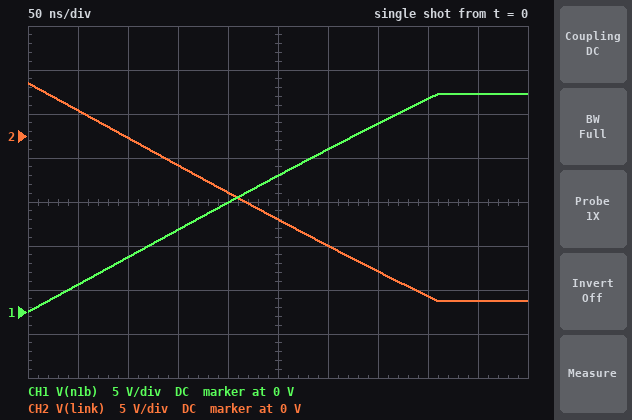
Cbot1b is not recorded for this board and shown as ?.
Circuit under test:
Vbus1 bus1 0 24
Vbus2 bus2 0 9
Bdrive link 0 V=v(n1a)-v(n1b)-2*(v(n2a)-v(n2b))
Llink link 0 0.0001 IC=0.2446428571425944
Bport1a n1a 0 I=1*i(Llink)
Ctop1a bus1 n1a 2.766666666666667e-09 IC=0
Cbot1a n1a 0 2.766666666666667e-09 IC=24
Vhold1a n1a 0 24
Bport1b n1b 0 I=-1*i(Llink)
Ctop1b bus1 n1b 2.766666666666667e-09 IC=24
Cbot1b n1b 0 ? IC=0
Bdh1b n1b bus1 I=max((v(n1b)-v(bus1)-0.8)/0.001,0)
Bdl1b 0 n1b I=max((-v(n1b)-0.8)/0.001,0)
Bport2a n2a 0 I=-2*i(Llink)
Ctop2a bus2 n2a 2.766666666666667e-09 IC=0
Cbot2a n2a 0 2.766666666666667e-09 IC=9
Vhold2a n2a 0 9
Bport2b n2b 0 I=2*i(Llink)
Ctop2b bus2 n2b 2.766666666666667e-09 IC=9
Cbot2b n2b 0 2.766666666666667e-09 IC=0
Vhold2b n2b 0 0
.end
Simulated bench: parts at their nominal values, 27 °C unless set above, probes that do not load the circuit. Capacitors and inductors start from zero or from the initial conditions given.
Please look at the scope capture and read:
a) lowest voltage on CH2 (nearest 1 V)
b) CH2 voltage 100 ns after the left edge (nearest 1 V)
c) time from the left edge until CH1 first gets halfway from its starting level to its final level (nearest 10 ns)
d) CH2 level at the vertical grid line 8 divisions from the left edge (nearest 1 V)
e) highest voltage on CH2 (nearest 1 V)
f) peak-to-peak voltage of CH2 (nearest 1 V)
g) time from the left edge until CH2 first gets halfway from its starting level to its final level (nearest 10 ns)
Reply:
-19 V
0 V
200 ns
-18 V
6 V
25 V
200 ns
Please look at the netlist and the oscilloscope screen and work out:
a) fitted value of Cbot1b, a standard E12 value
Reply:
1.2 nF
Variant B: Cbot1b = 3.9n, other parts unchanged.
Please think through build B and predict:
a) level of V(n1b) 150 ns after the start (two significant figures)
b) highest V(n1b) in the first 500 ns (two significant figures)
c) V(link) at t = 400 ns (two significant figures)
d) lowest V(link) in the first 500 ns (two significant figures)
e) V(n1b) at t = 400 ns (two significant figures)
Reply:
5.6 V
18 V
-8.8 V
-12 V
15 V
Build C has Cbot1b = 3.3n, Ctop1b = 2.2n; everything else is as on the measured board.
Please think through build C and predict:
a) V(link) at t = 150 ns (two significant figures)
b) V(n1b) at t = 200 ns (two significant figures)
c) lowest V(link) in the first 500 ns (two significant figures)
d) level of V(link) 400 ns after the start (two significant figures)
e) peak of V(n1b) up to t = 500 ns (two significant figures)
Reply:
-750 mV
9.0 V
-16 V
-12 V
22 V
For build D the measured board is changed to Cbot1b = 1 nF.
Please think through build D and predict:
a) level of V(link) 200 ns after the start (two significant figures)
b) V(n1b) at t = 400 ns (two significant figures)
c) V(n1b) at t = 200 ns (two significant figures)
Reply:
-7.1 V
25 V
13 V
